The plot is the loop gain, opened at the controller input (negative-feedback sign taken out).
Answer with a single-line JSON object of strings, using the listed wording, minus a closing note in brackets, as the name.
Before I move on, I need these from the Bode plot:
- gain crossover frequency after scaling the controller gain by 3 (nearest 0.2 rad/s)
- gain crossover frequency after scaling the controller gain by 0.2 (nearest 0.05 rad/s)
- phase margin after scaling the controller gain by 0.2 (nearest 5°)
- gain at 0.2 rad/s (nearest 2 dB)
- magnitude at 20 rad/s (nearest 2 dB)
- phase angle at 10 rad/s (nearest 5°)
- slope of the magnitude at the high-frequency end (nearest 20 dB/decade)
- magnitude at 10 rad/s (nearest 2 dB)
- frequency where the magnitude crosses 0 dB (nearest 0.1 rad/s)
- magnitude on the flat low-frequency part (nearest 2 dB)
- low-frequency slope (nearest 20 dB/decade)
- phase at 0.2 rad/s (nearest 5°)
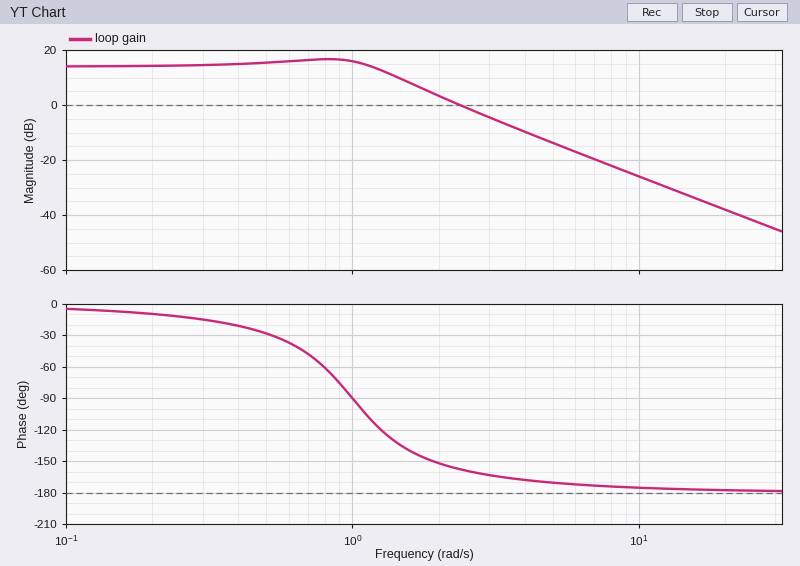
{"gain crossover frequency after scaling the controller gain by 3": "4.0 rad/s", "gain crossover frequency after scaling the controller gain by 0.2": "1.15 rad/s", "phase margin after scaling the controller gain by 0.2": "70°", "gain at 0.2 rad/s": "14 dB", "magnitude at 20 rad/s": "-38 dB", "phase angle at 10 rad/s": "-175°", "slope of the magnitude at the high-frequency end": "-40 dB/decade", "magnitude at 10 rad/s": "-26 dB", "frequency where the magnitude crosses 0 dB": "2.4 rad/s", "magnitude on the flat low-frequency part": "14 dB", "low-frequency slope": "0 dB/decade", "phase at 0.2 rad/s": "-10°"}
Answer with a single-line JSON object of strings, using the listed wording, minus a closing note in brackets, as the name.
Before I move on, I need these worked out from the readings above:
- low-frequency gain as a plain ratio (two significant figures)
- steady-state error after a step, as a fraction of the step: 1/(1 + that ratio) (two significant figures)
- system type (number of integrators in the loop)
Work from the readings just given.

{"low-frequency gain as a plain ratio": "5.0", "steady-state error after a step, as a fraction of the step: 1/(1 + that ratio)": "0.17", "system type": "0"}
